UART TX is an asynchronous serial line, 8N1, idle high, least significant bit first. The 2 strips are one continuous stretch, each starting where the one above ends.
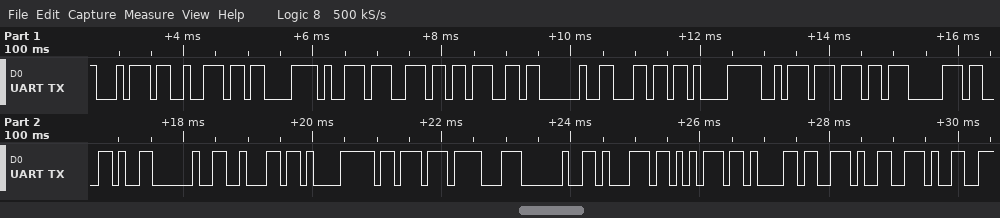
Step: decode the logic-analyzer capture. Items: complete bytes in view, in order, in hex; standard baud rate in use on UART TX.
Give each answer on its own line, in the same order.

74 72 C3 B9 6E 67 20 6C E1 BA B7 70 2C 20 62 E1 BB 8F 20 71 75 61 2E 2E
9600 baud
